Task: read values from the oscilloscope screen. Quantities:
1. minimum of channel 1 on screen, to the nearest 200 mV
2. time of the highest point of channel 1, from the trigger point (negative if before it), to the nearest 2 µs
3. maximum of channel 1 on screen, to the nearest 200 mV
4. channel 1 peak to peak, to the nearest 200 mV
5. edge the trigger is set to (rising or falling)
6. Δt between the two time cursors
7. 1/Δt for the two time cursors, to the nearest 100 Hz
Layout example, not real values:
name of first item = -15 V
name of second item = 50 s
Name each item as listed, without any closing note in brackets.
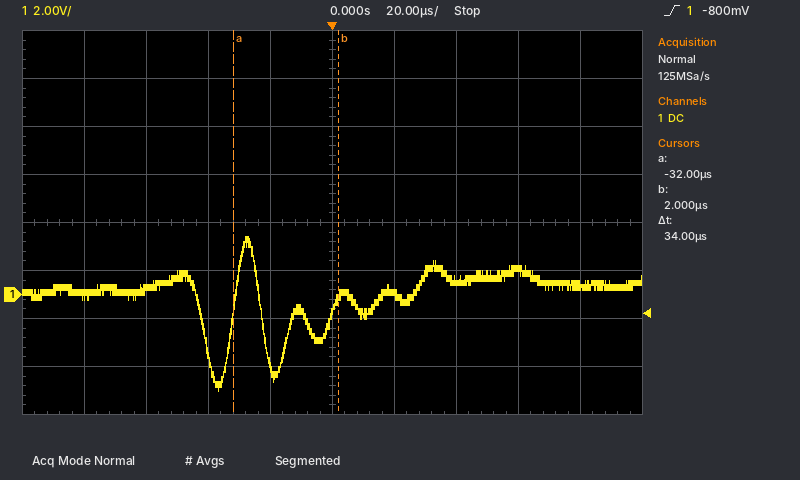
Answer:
minimum of channel 1 on screen, to the nearest 200 mV = -4.0 V
time of the highest point of channel 1, from the trigger point (negative if before it), to the nearest 2 µs = -28 µs
maximum of channel 1 on screen, to the nearest 200 mV = 2.4 V
channel 1 peak to peak, to the nearest 200 mV = 6.4 V
edge the trigger is set to = rising
Δt between the two time cursors = 34 µs
1/Δt for the two time cursors, to the nearest 100 Hz = 29.4 kHz
